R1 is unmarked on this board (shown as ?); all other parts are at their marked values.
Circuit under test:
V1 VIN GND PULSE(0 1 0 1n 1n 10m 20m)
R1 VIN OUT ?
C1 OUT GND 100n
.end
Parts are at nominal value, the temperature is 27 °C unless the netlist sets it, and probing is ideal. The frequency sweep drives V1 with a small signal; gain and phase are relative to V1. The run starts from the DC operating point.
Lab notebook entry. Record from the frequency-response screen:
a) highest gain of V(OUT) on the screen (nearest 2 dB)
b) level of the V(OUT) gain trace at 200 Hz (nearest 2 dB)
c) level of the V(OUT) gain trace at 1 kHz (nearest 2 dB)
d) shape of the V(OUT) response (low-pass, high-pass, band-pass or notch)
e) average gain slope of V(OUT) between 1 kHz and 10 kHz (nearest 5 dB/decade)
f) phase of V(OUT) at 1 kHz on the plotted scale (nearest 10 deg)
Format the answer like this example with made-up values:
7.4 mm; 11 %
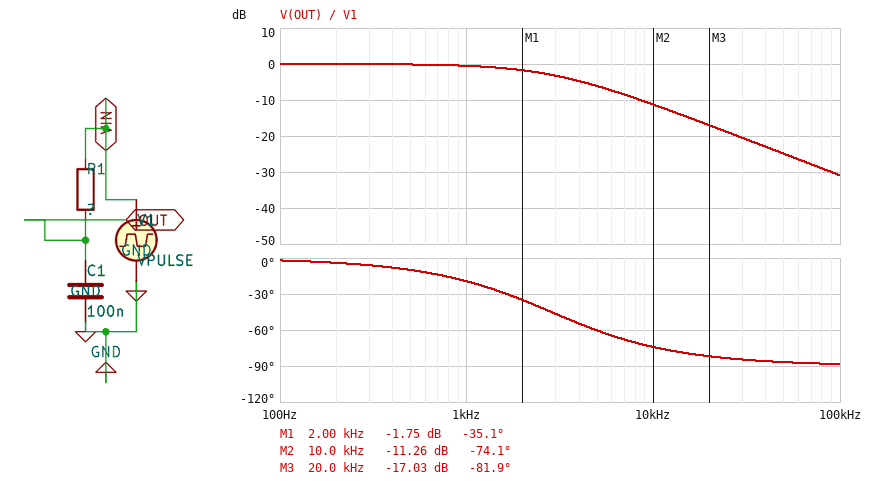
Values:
0 dB; 0 dB; 0 dB; low-pass; -10 dB/decade; -20 deg
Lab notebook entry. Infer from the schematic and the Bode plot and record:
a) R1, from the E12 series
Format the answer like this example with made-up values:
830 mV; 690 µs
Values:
560 Ω
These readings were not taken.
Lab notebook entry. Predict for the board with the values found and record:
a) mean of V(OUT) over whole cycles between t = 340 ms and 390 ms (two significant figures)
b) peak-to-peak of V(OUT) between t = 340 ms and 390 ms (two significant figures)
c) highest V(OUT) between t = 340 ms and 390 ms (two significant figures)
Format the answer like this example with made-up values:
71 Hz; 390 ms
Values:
500 mV; 1.0 V; 1.0 V
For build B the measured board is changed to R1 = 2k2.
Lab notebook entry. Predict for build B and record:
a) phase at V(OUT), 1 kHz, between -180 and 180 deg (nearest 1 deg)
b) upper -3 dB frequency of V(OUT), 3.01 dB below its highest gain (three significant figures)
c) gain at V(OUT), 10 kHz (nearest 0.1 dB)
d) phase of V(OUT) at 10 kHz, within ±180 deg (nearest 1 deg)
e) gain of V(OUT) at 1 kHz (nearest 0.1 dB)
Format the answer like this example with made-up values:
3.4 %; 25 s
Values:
-54 deg; 723 Hz; -22.8 dB; -86 deg; -4.6 dB
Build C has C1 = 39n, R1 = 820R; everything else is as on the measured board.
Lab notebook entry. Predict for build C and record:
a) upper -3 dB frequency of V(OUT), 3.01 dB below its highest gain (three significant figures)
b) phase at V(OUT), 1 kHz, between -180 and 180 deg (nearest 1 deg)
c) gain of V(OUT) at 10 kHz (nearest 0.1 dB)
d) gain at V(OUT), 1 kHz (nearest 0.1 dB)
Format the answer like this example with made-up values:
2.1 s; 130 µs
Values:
4.98 kHz; -11 deg; -7.0 dB; -0.2 dB
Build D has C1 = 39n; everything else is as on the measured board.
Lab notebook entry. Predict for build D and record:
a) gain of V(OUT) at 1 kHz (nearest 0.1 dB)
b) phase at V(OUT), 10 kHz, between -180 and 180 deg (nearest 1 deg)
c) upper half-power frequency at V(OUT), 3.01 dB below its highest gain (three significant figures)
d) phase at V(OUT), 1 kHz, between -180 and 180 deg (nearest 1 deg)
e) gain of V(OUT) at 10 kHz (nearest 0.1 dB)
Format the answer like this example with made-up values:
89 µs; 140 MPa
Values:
-0.1 dB; -54 deg; 7.29 kHz; -8 deg; -4.6 dB
